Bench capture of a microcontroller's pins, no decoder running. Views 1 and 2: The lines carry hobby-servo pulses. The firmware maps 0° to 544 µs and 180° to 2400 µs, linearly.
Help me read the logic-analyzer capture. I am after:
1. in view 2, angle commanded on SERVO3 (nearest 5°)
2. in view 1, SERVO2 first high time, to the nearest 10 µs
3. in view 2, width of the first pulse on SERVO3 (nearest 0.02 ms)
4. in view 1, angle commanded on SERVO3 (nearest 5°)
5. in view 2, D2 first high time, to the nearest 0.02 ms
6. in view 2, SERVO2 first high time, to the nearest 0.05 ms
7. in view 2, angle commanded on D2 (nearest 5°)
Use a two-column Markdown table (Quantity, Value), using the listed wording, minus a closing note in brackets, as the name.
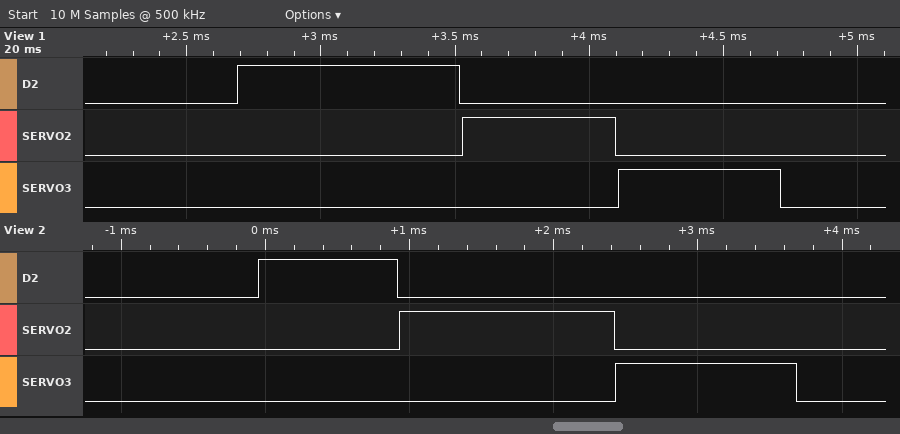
| Quantity | Value |
|---|---|
| in view 2, angle commanded on SERVO3 | 70° |
| in view 1, SERVO2 first high time, to the nearest 10 µs | 570 µs |
| in view 2, width of the first pulse on SERVO3 | 1.26 ms |
| in view 1, angle commanded on SERVO3 | 5° |
| in view 2, D2 first high time, to the nearest 0.02 ms | 0.96 ms |
| in view 2, SERVO2 first high time, to the nearest 0.05 ms | 1.50 ms |
| in view 2, angle commanded on D2 | 40° |
